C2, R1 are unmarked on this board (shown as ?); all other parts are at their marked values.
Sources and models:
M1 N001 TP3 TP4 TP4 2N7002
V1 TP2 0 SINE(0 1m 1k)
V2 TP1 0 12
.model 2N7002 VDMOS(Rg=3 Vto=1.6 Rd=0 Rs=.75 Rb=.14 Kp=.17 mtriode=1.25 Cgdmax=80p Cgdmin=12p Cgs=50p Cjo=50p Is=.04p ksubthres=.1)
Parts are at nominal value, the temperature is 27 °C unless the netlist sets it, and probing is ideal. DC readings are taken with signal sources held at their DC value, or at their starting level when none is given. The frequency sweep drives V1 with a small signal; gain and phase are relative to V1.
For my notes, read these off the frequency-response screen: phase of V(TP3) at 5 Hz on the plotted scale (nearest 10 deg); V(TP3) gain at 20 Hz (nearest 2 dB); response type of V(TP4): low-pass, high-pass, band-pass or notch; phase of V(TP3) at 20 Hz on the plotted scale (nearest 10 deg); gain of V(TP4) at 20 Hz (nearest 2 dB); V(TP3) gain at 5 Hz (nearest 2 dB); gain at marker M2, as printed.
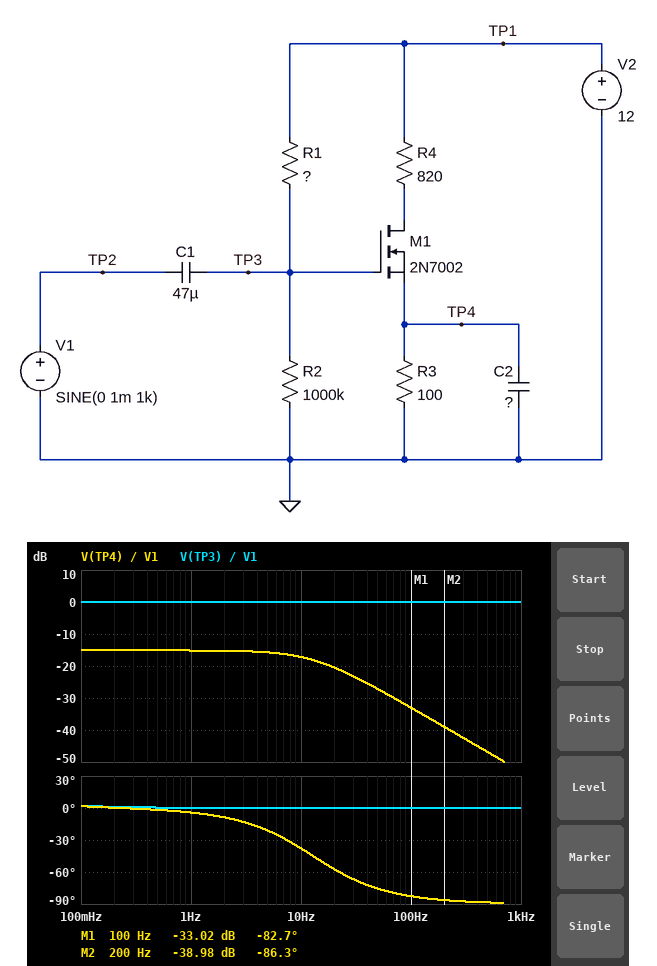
0 deg
0 dB
low-pass
0 deg
-20 dB
0 dB
-38.98 dB
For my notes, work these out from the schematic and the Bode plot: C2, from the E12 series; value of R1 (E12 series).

150 µF
6.8 MΩ
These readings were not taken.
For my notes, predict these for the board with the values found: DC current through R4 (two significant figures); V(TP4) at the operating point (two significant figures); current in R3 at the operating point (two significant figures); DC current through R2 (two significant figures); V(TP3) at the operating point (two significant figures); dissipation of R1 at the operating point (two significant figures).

130 µA
13 mV
130 µA
1.5 µA
1.5 V
16 µW
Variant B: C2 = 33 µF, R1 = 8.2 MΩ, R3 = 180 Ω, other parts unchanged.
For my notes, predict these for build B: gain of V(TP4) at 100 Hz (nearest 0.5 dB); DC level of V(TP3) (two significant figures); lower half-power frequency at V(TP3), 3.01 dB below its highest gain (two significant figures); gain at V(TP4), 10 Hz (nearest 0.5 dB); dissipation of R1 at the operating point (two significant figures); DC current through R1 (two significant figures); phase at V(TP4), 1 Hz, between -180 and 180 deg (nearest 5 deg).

-54.0 dB
1.3 V
3.8 mHz
-43.0 dB
14 µW
1.3 µA
0 deg
